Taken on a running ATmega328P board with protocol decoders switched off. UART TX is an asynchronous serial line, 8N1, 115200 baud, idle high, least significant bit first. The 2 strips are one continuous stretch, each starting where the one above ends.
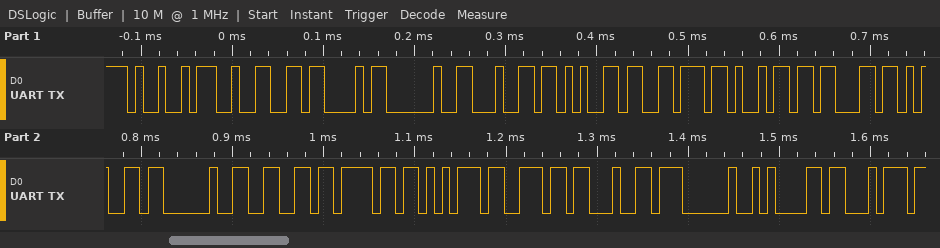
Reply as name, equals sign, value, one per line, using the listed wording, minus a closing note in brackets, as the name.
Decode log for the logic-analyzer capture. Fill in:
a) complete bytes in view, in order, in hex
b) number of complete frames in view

complete bytes in view, in order, in hex = 0x49 0x32 0x43 0x20 0x64 0x65 0x76 0x69 0x63 0x65 0x20 0x66 0x6F 0x75 0x6E 0x64 0x20 0x61 0x74
number of complete frames in view = 19
